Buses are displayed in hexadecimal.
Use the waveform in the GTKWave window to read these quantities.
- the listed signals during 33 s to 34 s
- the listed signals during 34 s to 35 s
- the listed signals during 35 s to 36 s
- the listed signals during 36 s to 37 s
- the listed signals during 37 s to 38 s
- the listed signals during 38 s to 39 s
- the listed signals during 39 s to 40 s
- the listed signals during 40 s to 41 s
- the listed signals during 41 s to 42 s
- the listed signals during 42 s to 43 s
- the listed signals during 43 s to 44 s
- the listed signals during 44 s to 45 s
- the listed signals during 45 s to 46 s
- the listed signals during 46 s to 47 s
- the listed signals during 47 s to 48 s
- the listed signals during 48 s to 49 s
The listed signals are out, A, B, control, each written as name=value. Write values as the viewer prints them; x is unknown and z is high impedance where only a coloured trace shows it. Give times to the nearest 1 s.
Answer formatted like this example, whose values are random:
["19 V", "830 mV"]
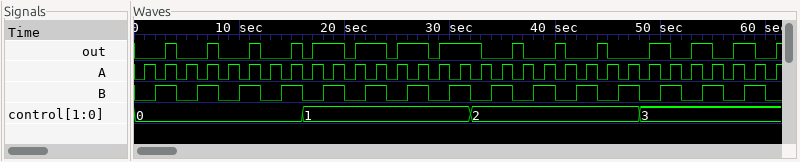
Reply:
["out=0, A=1, B=0, control=2", "out=0, A=0, B=1, control=2", "out=0, A=1, B=1, control=2", "out=1, A=0, B=0, control=2", "out=0, A=1, B=0, control=2", "out=0, A=0, B=1, control=2", "out=0, A=1, B=1, control=2", "out=1, A=0, B=0, control=2", "out=0, A=1, B=0, control=2", "out=0, A=0, B=1, control=2", "out=0, A=1, B=1, control=2", "out=1, A=0, B=0, control=2", "out=0, A=1, B=0, control=2", "out=0, A=0, B=1, control=2", "out=0, A=1, B=1, control=2", "out=0, A=0, B=0, control=3"]
